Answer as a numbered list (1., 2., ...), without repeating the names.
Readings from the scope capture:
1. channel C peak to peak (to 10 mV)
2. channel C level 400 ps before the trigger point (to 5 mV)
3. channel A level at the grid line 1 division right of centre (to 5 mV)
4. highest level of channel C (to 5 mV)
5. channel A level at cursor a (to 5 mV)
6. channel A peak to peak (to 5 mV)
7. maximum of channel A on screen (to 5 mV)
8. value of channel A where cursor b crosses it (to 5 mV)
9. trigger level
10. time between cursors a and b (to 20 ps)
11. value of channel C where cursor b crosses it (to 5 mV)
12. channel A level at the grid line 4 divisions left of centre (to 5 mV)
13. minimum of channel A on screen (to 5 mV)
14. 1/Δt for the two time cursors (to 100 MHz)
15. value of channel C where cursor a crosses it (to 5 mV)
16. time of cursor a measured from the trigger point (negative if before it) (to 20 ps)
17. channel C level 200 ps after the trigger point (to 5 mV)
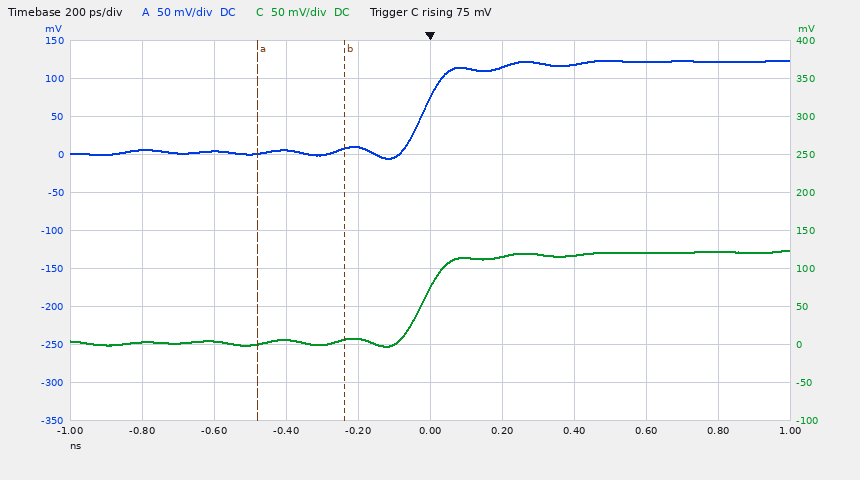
1. 130 mV
2. 5 mV
3. 115 mV
4. 125 mV
5. 0 mV
6. 130 mV
7. 125 mV
8. 10 mV
9. 75 mV
10. 240 ps
11. 5 mV
12. 5 mV
13. -5 mV
14. 4.2 GHz
15. 0 mV
16. -480 ps
17. 115 mV
